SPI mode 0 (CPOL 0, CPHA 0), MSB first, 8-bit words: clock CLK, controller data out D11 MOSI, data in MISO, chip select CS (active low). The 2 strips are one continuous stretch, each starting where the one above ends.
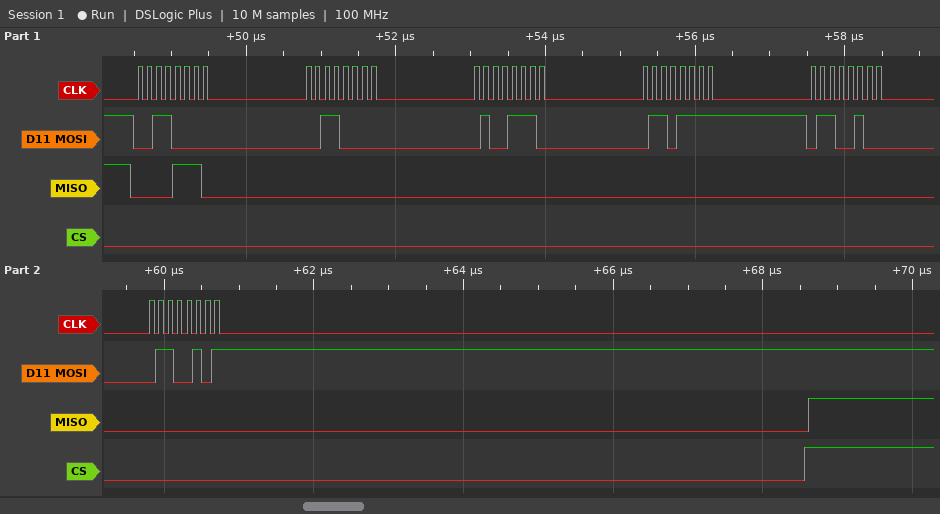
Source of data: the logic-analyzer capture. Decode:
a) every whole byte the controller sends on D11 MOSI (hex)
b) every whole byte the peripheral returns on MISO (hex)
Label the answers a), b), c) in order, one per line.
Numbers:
a) 30 30 4E 6F 64 65
b) 0E 00 00 00 00 00
